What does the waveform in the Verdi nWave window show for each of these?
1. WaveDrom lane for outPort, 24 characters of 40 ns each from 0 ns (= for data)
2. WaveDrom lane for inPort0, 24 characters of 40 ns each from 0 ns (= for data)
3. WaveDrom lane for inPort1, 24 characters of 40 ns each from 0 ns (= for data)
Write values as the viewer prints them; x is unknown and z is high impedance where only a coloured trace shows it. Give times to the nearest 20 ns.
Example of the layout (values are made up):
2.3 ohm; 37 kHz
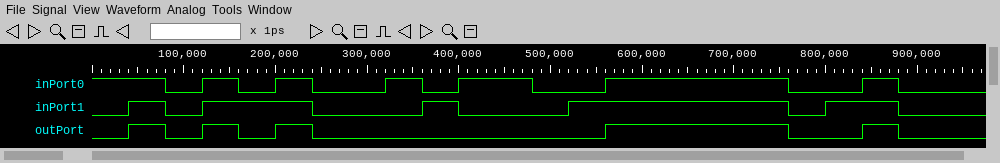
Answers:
{name: 'outPort', wave: '0101010.......1....0.10.'}; {name: 'inPort0', wave: '1.01010.101.0.1....0.10.'}; {name: 'inPort1', wave: '0101..0..10..1.....01.0.'}
